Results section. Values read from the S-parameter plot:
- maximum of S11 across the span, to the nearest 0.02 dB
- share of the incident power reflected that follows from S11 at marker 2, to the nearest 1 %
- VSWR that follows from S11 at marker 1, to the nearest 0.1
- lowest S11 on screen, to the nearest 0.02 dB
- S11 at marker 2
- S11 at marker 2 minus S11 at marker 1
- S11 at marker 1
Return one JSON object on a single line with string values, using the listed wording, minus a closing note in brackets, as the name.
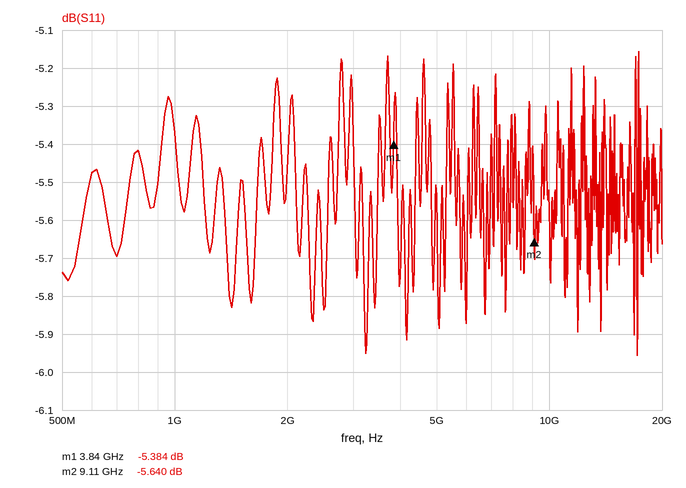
{"maximum of S11 across the span, to the nearest 0.02 dB": "-5.16 dB", "share of the incident power reflected that follows from S11 at marker 2, to the nearest 1 %": "27 %", "VSWR that follows from S11 at marker 1, to the nearest 0.1": "3.3", "lowest S11 on screen, to the nearest 0.02 dB": "-5.96 dB", "S11 at marker 2": "-5.640 dB", "S11 at marker 2 minus S11 at marker 1": "-0.256 dB", "S11 at marker 1": "-5.384 dB"}
